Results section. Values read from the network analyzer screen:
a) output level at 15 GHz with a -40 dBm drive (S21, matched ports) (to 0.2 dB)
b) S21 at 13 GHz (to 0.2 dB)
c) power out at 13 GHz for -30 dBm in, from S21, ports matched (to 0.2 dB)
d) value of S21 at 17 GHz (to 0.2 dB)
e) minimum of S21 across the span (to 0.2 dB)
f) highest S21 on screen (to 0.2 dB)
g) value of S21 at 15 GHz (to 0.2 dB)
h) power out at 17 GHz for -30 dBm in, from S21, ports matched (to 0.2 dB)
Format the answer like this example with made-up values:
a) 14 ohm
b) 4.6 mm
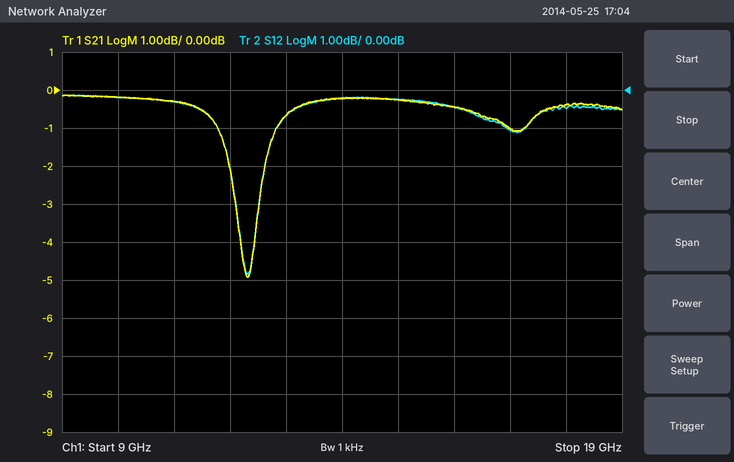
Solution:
a) -40.2 dBm
b) -0.6 dB
c) -30.6 dBm
d) -1.0 dB
e) -5.0 dB
f) -0.2 dB
g) -0.2 dB
h) -31.0 dBm
